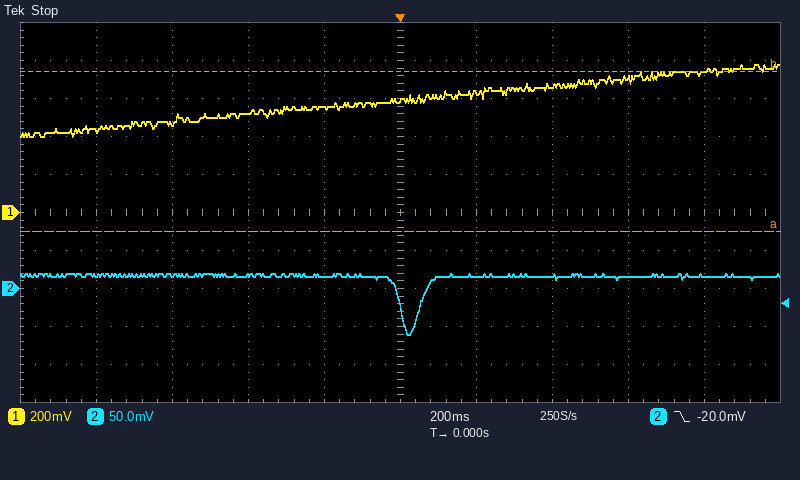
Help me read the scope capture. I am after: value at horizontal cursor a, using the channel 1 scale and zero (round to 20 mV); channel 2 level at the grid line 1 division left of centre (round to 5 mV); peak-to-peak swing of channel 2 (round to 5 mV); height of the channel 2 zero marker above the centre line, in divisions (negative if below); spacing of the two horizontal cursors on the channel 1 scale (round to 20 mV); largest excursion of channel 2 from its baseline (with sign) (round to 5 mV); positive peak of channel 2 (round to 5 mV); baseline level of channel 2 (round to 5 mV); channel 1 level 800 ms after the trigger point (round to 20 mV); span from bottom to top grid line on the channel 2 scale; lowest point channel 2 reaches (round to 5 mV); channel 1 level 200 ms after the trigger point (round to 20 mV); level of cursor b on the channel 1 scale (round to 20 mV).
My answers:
-100 mV
15 mV
80 mV
-2.0 div
840 mV
-75 mV
20 mV
15 mV
740 mV
500 mV
-60 mV
620 mV
740 mV
